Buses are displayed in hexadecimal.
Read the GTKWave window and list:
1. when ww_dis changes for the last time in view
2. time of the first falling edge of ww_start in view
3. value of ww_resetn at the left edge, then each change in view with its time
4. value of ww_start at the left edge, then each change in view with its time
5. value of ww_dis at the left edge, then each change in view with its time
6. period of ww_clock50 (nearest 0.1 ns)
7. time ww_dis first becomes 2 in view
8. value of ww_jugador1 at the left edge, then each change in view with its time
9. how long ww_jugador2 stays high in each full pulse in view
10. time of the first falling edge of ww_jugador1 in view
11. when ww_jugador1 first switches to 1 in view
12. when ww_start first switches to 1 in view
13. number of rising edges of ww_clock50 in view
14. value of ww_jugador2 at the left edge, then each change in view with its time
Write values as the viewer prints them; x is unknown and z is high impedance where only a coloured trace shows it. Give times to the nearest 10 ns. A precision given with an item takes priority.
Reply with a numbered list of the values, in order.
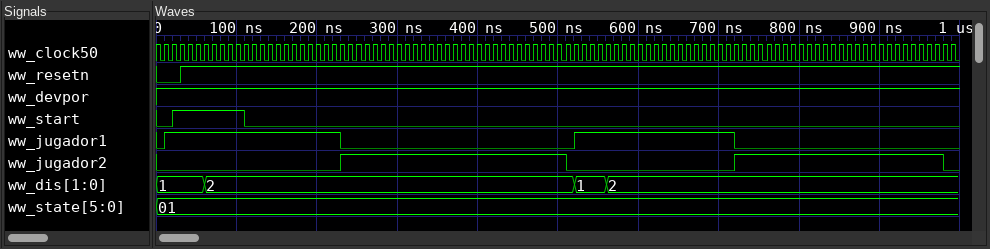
1. 560 ns
2. 110 ns
3. 0, 1 at 30 ns
4. 0, 1 at 20 ns, 0 at 110 ns
5. 1, 2 at 60 ns, 1 at 520 ns, 2 at 560 ns
6. 10 ns
7. 60 ns
8. 0, 1 at 10 ns, 0 at 230 ns, 1 at 520 ns, 0 at 720 ns
9. 280 ns, 260 ns
10. 230 ns
11. 10 ns
12. 20 ns
13. 99
14. 0, 1 at 230 ns, 0 at 510 ns, 1 at 720 ns, 0 at 980 ns
